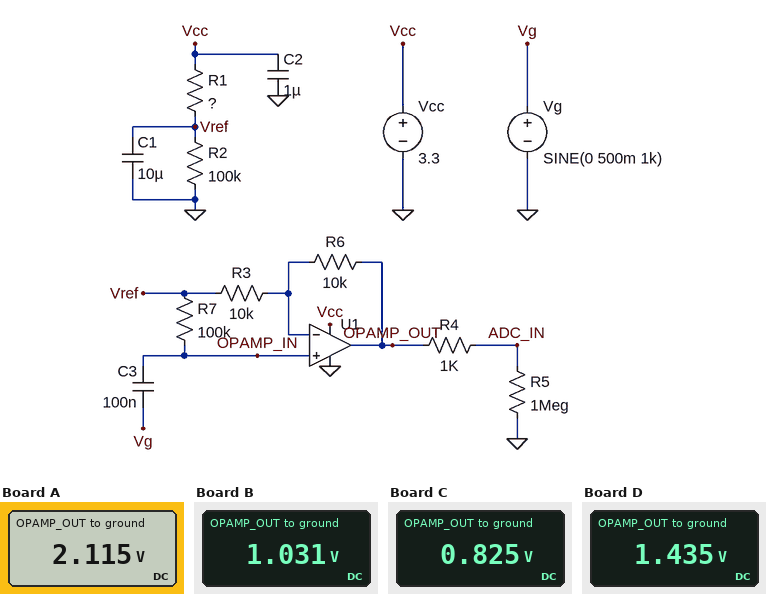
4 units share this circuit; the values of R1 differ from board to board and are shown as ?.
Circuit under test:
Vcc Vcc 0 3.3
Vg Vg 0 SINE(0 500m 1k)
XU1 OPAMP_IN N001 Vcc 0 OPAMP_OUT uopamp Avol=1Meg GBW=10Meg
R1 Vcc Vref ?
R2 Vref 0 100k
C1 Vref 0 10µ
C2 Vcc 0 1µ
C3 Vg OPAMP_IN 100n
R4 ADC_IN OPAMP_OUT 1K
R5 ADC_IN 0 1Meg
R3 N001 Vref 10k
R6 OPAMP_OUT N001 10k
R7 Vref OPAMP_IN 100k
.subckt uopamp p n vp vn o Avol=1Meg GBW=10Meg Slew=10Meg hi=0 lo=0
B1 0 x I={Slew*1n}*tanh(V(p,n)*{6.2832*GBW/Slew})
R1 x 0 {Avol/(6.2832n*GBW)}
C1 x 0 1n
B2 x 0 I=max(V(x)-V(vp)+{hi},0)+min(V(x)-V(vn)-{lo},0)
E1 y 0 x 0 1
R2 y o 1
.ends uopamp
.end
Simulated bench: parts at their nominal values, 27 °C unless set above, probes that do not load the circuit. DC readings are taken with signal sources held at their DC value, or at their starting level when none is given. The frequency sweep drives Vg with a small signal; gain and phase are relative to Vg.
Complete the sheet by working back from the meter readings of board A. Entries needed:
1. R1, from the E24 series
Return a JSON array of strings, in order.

["56 kΩ"]
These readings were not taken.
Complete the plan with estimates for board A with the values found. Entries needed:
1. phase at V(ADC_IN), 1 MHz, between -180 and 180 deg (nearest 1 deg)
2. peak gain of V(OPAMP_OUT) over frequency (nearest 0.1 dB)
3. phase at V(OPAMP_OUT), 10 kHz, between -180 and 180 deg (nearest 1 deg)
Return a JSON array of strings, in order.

["-11 deg", "6.0 dB", "0 deg"]
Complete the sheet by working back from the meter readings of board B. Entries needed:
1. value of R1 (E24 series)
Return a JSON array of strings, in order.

["220 kΩ"]
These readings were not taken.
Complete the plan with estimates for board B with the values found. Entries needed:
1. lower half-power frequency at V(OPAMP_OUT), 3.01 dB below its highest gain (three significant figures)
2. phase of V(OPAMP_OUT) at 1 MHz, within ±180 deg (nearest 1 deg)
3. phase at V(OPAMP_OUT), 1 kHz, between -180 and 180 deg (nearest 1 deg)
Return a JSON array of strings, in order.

["17.6 Hz", "-11 deg", "1 deg"]
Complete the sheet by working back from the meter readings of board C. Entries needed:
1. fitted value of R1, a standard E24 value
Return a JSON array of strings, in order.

["300 kΩ"]
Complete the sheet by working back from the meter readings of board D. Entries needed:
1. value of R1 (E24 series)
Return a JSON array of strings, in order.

["130 kΩ"]
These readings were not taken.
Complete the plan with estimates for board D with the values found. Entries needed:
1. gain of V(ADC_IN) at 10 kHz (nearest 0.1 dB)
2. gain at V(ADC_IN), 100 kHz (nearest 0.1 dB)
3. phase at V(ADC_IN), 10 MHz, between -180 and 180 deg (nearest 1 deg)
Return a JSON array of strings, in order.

["6.0 dB", "6.0 dB", "-63 deg"]
